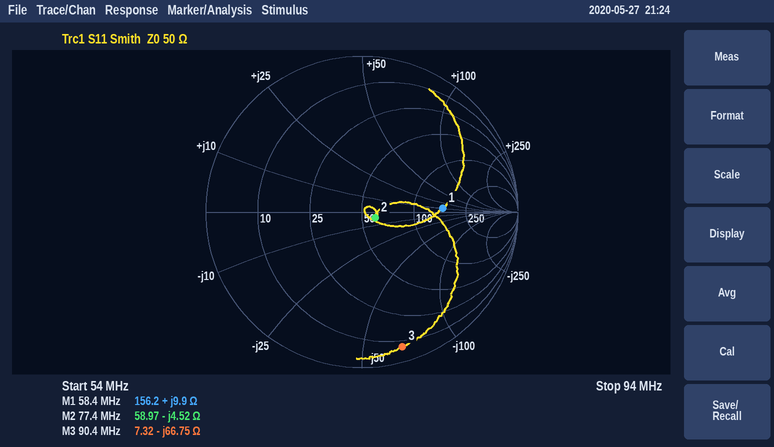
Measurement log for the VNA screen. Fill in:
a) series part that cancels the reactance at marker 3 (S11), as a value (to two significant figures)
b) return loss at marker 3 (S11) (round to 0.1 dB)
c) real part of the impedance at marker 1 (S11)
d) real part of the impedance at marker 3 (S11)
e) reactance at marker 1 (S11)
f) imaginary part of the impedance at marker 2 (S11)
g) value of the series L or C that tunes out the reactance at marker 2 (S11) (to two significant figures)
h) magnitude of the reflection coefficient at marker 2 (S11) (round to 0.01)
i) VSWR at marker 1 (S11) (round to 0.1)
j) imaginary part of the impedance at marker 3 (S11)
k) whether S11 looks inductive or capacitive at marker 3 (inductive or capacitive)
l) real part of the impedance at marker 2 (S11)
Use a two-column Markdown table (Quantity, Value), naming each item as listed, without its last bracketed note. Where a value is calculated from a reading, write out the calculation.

| Quantity | Value |
|---|---|
| series part that cancels the reactance at marker 3 (S11), as a value | L = 66.75 Ω/(2π × 90.4 MHz) ≈ 118 nH, so 120 nH to two significant figures |
| return loss at marker 3 (S11) | 0.9 dB |
| real part of the impedance at marker 1 | 156.2 Ω |
| real part of the impedance at marker 3 | 7.32 Ω |
| reactance at marker 1 | +9.9 Ω |
| imaginary part of the impedance at marker 2 | -4.52 Ω |
| value of the series L or C that tunes out the reactance at marker 2 (S11) | L = 4.52 Ω/(2π × 77.4 MHz) ≈ 9.3 nH |
| magnitude of the reflection coefficient at marker 2 (S11) | 0.09 |
| VSWR at marker 1 (S11) | 3.1 |
| imaginary part of the impedance at marker 3 | -66.75 Ω |
| whether S11 looks inductive or capacitive at marker 3 | capacitive |
| real part of the impedance at marker 2 | 58.97 Ω |
